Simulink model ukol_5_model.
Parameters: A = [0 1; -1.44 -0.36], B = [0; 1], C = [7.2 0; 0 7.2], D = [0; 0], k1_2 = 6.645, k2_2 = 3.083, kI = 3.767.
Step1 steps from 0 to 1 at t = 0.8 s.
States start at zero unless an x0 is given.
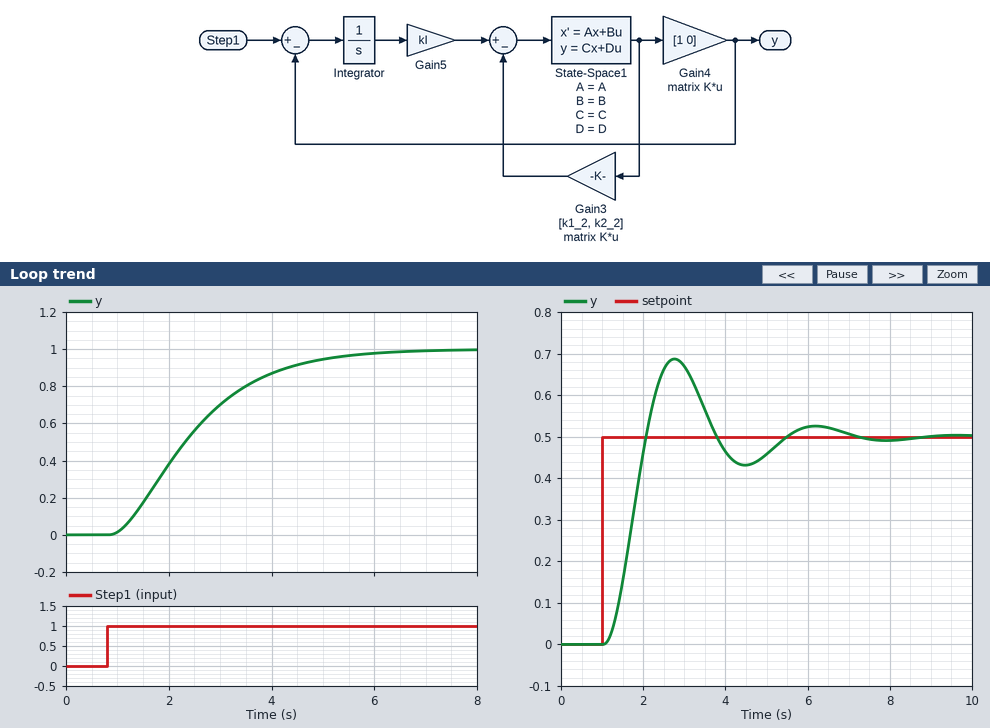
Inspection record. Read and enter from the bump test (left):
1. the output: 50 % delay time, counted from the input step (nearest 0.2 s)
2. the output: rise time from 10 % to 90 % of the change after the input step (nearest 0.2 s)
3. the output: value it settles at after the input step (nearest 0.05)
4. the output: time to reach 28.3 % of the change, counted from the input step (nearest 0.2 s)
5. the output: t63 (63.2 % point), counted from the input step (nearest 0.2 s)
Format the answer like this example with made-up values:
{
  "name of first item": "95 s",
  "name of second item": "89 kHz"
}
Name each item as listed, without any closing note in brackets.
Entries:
{
  "the output: 50 % delay time, counted from the input step": "1.6 s",
  "the output: rise time from 10 % to 90 % of the change after the input step": "3.0 s",
  "the output: value it settles at after the input step": "1.00",
  "the output: time to reach 28.3 % of the change, counted from the input step": "1.0 s",
  "the output: t63 (63.2 % point), counted from the input step": "2.0 s"
}
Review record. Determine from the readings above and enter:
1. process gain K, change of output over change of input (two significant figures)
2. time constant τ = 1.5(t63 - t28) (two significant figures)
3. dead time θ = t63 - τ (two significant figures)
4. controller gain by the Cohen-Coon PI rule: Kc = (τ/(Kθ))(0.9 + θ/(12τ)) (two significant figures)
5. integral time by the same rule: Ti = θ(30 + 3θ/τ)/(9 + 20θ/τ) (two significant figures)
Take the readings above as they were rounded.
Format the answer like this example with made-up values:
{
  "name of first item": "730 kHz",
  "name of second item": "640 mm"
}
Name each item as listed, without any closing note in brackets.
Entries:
{
  "process gain K, change of output over change of input": "1.0",
  "time constant τ = 1.5(t63 - t28)": "1.5 s",
  "dead time θ = t63 - τ": "0.50 s",
  "controller gain by the Cohen-Coon PI rule: Kc = (τ/(Kθ))(0.9 + θ/(12τ))": "2.8",
  "integral time by the same rule: Ti = θ(30 + 3θ/τ)/(9 + 20θ/τ)": "0.99 s"
}
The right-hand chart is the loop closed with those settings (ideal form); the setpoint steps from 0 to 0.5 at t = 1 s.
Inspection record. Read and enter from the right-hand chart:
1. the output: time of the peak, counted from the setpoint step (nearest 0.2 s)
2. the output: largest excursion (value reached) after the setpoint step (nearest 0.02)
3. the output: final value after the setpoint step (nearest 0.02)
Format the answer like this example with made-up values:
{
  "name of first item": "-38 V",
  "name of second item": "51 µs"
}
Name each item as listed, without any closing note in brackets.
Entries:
{
  "the output: time of the peak, counted from the setpoint step": "1.8 s",
  "the output: largest excursion (value reached) after the setpoint step": "0.68",
  "the output: final value after the setpoint step": "0.50"
}
